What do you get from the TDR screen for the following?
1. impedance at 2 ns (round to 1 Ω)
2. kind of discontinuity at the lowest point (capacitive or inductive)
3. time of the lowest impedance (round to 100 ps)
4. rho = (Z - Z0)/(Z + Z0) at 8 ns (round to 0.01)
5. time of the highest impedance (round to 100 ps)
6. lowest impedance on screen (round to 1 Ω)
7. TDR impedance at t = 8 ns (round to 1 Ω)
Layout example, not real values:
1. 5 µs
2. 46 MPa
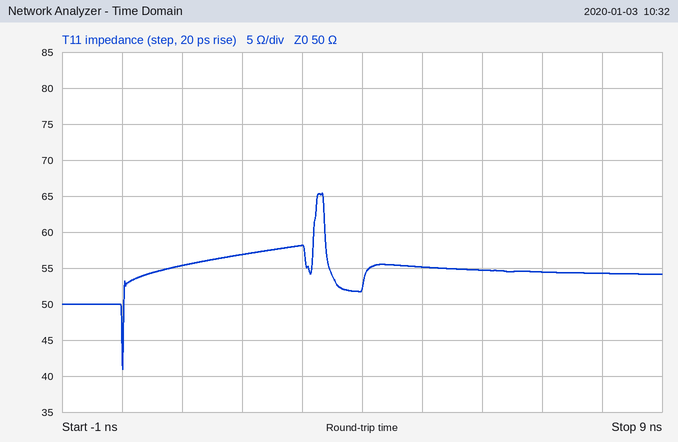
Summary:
1. 57 Ω
2. capacitive
3. 0.0 ns
4. +0.04
5. 3.3 ns
6. 41 Ω
7. 54 Ω
